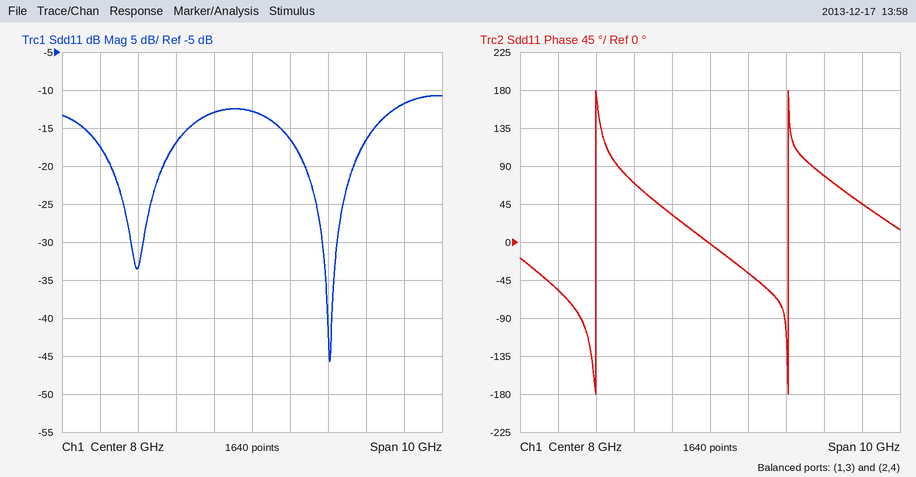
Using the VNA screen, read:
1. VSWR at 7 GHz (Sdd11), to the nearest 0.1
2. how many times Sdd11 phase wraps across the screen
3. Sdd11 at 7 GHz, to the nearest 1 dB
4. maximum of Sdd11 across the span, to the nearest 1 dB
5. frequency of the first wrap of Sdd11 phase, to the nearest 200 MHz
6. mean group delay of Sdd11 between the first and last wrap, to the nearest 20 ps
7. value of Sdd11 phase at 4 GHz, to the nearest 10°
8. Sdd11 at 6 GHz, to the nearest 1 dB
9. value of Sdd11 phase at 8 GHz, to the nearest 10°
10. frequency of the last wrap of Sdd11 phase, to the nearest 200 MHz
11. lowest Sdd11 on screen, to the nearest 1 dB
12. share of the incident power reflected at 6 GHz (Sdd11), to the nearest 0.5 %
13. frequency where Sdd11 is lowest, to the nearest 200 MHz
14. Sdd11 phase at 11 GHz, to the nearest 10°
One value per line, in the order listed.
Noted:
1.6
2
-13 dB
-11 dB
5.0 GHz
200 ps
-60°
-17 dB
0°
10.0 GHz
-46 dB
2.0 %
10.0 GHz
80°
